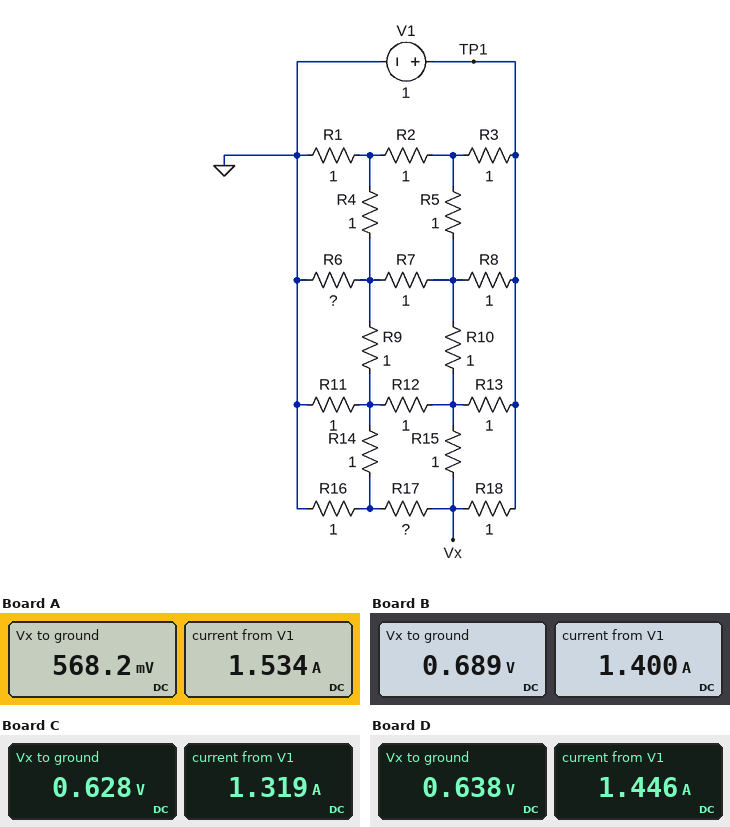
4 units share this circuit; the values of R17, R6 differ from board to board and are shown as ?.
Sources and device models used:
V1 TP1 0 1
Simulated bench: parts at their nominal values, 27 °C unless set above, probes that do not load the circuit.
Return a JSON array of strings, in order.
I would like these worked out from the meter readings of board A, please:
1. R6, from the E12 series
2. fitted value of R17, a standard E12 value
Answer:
["0.47 Ω", "0.33 Ω"]
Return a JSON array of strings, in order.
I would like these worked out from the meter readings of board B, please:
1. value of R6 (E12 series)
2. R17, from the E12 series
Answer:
["0.39 Ω", "1.5 Ω"]
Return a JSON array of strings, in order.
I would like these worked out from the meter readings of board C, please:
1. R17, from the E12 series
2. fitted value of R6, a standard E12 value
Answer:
["0.56 Ω", "2.2 Ω"]
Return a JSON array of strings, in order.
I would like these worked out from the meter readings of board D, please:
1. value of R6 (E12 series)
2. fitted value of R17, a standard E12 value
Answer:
["0.47 Ω", "0.82 Ω"]
